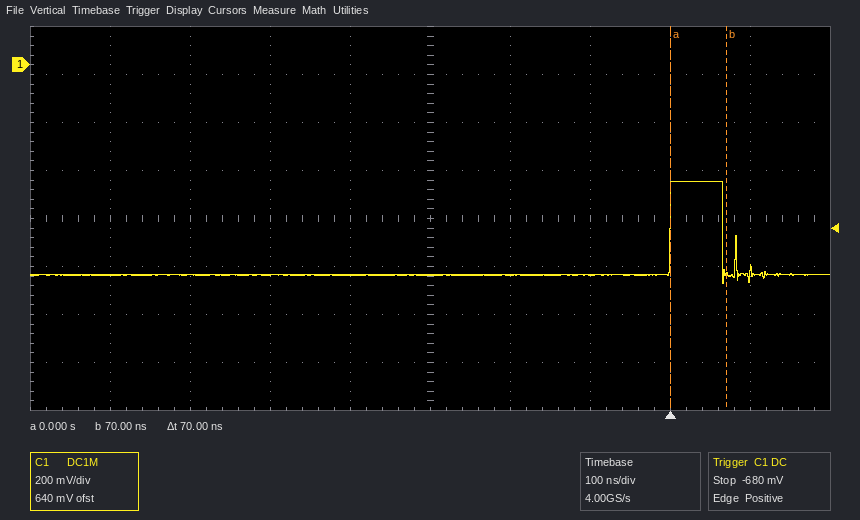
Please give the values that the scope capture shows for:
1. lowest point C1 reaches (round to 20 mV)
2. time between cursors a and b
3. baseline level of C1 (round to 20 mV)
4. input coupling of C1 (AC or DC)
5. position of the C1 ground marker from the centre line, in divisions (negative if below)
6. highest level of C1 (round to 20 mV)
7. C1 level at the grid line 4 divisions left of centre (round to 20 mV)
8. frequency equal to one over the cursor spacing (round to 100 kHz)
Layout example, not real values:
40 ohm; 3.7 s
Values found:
-920 mV; 70 ns; -880 mV; DC; +3.2 div; -480 mV; -880 mV; 14.3 MHz
